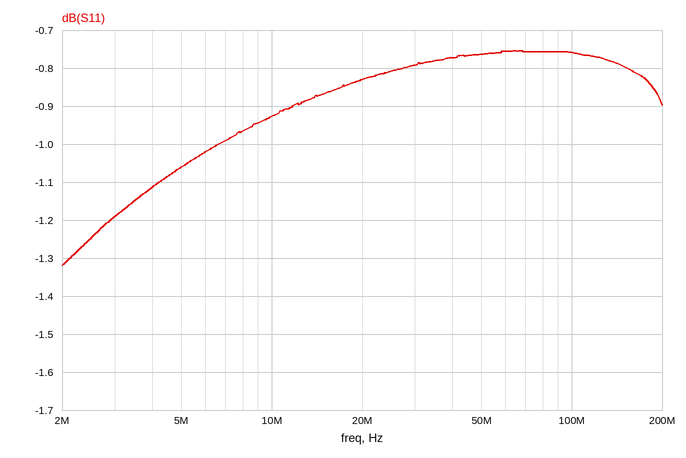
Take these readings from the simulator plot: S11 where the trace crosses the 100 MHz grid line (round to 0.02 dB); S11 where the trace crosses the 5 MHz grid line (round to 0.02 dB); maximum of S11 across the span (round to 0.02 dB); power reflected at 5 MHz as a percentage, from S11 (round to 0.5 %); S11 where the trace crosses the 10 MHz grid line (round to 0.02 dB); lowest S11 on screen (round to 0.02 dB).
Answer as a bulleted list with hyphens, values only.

- -0.76 dB
- -1.06 dB
- -0.76 dB
- 78.5 %
- -0.92 dB
- -1.32 dB
